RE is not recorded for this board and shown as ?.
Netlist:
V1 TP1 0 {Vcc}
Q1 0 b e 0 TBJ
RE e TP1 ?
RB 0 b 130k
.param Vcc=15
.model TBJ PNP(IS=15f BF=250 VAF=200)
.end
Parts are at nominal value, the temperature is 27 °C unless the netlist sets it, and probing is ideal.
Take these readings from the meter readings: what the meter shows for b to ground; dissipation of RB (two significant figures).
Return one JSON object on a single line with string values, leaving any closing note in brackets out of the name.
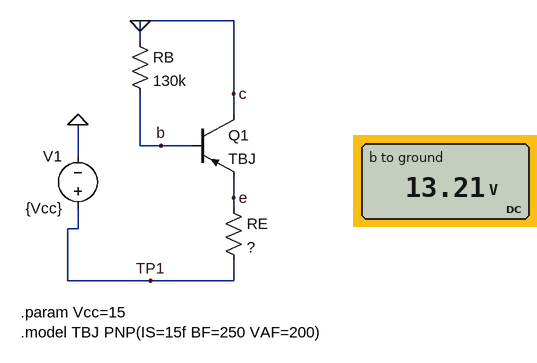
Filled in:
{"what the meter shows for b to ground": "13.21 V", "dissipation of RB": "1.3 mW"}
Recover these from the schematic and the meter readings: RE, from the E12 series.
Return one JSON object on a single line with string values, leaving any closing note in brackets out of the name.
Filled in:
{"RE, from the E12 series": "39 Ω"}
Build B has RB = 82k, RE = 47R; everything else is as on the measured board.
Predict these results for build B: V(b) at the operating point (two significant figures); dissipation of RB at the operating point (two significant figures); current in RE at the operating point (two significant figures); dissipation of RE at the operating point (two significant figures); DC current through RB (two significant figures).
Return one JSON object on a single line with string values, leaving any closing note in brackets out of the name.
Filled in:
{"V(b) at the operating point": "12 V", "dissipation of RB at the operating point": "1.9 mW", "current in RE at the operating point": "40 mA", "dissipation of RE at the operating point": "76 mW", "DC current through RB": "150 µA"}
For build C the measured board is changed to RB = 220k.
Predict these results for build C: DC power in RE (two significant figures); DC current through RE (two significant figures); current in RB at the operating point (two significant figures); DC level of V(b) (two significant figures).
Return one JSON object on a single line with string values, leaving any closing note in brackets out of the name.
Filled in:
{"DC power in RE": "11 mW", "DC current through RE": "17 mA", "current in RB at the operating point": "62 µA", "DC level of V(b)": "14 V"}
